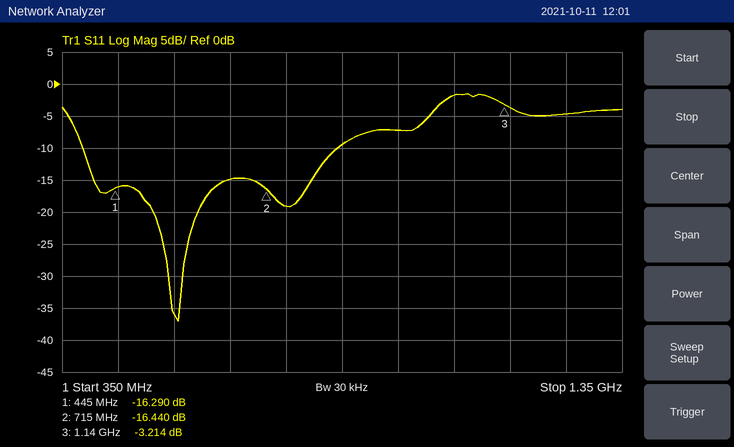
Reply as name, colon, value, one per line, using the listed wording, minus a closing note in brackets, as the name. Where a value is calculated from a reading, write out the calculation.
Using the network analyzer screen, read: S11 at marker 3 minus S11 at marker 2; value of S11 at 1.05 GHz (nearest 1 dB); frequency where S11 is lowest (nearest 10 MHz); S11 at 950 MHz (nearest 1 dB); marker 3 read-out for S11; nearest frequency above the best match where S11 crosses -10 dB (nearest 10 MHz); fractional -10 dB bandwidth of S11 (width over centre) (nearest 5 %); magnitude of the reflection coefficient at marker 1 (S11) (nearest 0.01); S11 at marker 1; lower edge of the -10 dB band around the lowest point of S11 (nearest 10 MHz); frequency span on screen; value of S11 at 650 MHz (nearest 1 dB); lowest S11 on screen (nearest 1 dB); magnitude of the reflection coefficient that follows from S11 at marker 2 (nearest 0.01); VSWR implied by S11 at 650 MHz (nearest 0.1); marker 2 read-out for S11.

S11 at marker 3 minus S11 at marker 2: -3.214 − (-16.44) = 13.226 dB
value of S11 at 1.05 GHz: -2 dB
frequency where S11 is lowest: 560 MHz
S11 at 950 MHz: -7 dB
marker 3 read-out for S11: -3.214 dB
nearest frequency above the best match where S11 crosses -10 dB: 840 MHz
fractional -10 dB bandwidth of S11 (width over centre): 450 MHz / 615 MHz ≈ 73.2 %, so 75 % to the nearest 5 %
magnitude of the reflection coefficient at marker 1 (S11): 10^(-16.29/20) ≈ 0.15
S11 at marker 1: -16.290 dB
lower edge of the -10 dB band around the lowest point of S11: 390 MHz
frequency span on screen: 1 GHz
value of S11 at 650 MHz: -15 dB
lowest S11 on screen: -37 dB
magnitude of the reflection coefficient that follows from S11 at marker 2: 10^(-16.44/20) ≈ 0.15
VSWR implied by S11 at 650 MHz: |Γ| = 10^(-15/20) = 0.1778; VSWR = (1 + 0.1778)/(1 − 0.1778) ≈ 1.4
marker 2 read-out for S11: -16.440 dB
